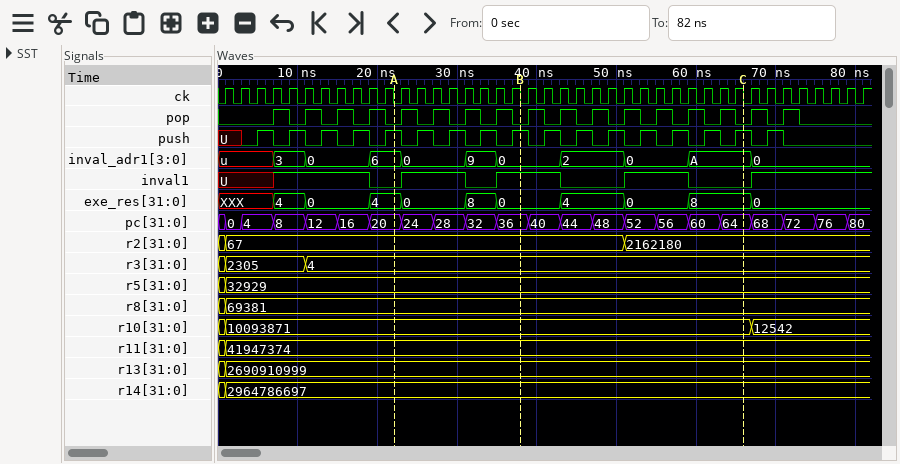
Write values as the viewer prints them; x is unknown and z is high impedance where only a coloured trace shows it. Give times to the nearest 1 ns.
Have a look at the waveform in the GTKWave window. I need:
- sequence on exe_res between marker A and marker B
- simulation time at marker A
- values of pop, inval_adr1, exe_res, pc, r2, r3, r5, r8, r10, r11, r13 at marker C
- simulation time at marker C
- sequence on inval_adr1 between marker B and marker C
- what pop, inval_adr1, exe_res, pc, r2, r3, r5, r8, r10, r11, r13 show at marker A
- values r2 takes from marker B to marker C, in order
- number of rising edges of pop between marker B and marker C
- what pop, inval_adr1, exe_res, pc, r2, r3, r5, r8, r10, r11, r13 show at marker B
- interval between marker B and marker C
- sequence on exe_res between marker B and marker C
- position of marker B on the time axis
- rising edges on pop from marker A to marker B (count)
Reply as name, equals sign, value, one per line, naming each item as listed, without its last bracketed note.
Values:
sequence on exe_res between marker A and marker B = 4, 0, 8, 0
simulation time at marker A = 22 ns
values of pop, inval_adr1, exe_res, pc, r2, r3, r5, r8, r10, r11, r13 at marker C = pop=0, inval_adr1=A, exe_res=8, pc=64, r2=2162180, r3=4, r5=32929, r8=69381, r10=10093871, r11=41947374, r13=2690910999
simulation time at marker C = 66 ns
sequence on inval_adr1 between marker B and marker C = 0, 2, 0, A
what pop, inval_adr1, exe_res, pc, r2, r3, r5, r8, r10, r11, r13 show at marker A = pop=0, inval_adr1=6, exe_res=4, pc=20, r2=67, r3=4, r5=32929, r8=69381, r10=10093871, r11=41947374, r13=2690910999
values r2 takes from marker B to marker C, in order = 67, 2162180
number of rising edges of pop between marker B and marker C = 7
what pop, inval_adr1, exe_res, pc, r2, r3, r5, r8, r10, r11, r13 show at marker B = pop=0, inval_adr1=0, exe_res=0, pc=36, r2=67, r3=4, r5=32929, r8=69381, r10=10093871, r11=41947374, r13=2690910999
interval between marker B and marker C = 28 ns
sequence on exe_res between marker B and marker C = 0, 4, 0, 8
position of marker B on the time axis = 38 ns
rising edges on pop from marker A to marker B = 4
